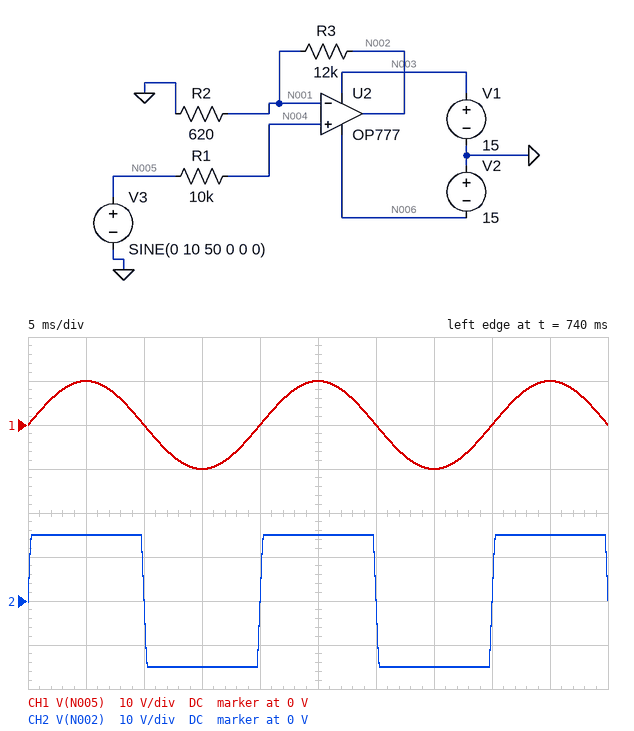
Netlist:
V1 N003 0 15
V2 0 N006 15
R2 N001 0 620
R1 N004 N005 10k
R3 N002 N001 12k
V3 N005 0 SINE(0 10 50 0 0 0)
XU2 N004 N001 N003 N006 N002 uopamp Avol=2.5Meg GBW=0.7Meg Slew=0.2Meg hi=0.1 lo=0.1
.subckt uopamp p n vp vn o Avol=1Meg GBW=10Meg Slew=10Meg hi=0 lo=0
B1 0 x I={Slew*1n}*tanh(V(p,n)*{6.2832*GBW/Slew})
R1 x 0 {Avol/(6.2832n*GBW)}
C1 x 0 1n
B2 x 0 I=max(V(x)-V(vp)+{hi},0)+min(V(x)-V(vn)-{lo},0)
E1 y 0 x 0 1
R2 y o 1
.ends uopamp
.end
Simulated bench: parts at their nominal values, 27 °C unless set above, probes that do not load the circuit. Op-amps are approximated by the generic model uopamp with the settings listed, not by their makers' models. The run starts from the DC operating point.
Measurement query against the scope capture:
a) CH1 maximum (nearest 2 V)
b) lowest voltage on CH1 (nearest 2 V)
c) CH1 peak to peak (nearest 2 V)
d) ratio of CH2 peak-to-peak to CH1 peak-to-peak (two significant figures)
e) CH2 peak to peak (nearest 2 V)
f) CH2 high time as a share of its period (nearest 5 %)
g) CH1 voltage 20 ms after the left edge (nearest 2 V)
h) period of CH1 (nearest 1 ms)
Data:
10 V
-10 V
20 V
1.5
30 V
50 %
0 V
20 ms
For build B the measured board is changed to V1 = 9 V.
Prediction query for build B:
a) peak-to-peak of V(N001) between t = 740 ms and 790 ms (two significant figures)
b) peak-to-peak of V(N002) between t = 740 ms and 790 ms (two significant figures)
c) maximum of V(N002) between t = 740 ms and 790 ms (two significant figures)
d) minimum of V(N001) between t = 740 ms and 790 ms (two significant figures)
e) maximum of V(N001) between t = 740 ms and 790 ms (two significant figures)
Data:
1.2 V
24 V
8.9 V
-730 mV
440 mV
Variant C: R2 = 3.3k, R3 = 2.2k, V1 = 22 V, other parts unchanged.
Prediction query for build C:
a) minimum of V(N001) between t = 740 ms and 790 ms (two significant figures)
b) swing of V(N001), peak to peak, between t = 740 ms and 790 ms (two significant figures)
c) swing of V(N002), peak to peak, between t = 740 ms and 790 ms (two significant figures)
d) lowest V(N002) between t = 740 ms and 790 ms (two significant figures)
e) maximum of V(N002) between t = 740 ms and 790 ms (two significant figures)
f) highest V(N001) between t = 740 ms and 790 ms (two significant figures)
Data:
-8.9 V
19 V
32 V
-15 V
17 V
10 V
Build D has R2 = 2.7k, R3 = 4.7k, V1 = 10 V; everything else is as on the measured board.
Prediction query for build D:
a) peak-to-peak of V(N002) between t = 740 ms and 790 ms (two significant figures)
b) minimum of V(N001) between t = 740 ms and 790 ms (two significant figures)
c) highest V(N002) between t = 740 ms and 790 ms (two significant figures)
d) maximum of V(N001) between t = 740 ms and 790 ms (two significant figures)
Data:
25 V
-5.4 V
9.9 V
3.6 V
